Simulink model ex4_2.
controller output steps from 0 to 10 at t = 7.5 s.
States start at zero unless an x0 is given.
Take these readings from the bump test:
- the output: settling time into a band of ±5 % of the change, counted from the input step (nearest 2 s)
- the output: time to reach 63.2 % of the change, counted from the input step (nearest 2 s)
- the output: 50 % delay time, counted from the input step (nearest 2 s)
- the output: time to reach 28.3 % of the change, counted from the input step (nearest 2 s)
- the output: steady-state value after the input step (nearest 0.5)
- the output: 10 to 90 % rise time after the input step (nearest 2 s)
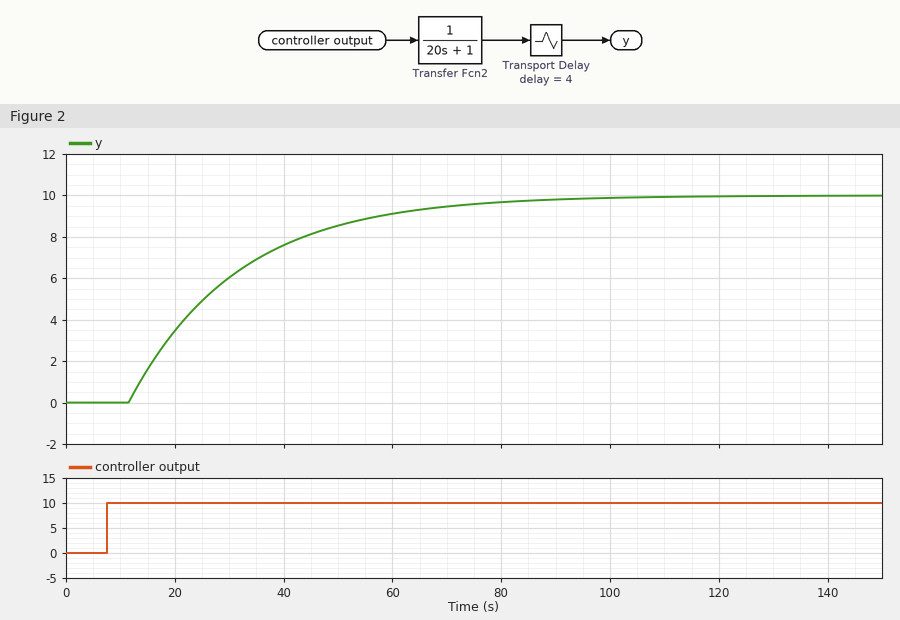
64 s
24 s
18 s
10 s
10.0
44 s
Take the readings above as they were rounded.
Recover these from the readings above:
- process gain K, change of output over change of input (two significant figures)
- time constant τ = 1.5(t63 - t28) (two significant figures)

1.0
21 s
